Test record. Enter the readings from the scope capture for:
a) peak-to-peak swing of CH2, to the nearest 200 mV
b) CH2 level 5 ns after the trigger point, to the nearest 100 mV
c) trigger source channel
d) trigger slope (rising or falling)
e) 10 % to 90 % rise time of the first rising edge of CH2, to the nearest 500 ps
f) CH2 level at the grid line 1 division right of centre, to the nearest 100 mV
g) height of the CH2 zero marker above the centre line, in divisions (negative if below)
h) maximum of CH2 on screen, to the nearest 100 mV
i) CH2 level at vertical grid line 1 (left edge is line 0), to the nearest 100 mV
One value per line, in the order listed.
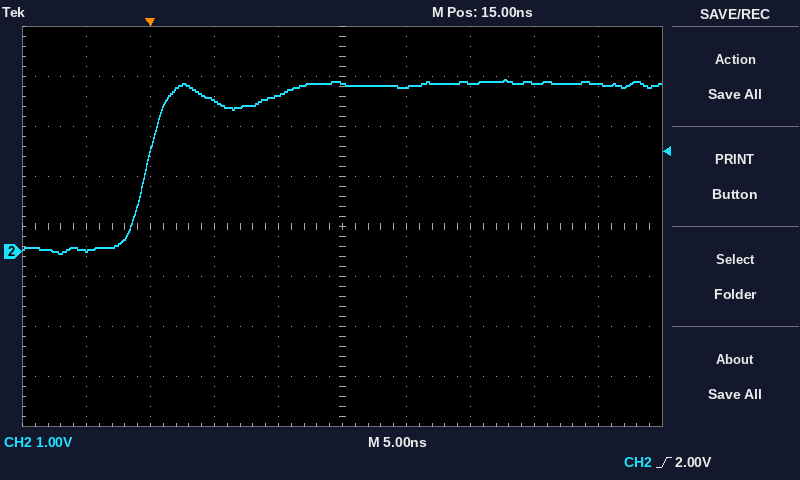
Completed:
3.4 V
3.0 V
CH2
rising
3.0 ns
3.3 V
-0.5 div
3.4 V
0.0 V
